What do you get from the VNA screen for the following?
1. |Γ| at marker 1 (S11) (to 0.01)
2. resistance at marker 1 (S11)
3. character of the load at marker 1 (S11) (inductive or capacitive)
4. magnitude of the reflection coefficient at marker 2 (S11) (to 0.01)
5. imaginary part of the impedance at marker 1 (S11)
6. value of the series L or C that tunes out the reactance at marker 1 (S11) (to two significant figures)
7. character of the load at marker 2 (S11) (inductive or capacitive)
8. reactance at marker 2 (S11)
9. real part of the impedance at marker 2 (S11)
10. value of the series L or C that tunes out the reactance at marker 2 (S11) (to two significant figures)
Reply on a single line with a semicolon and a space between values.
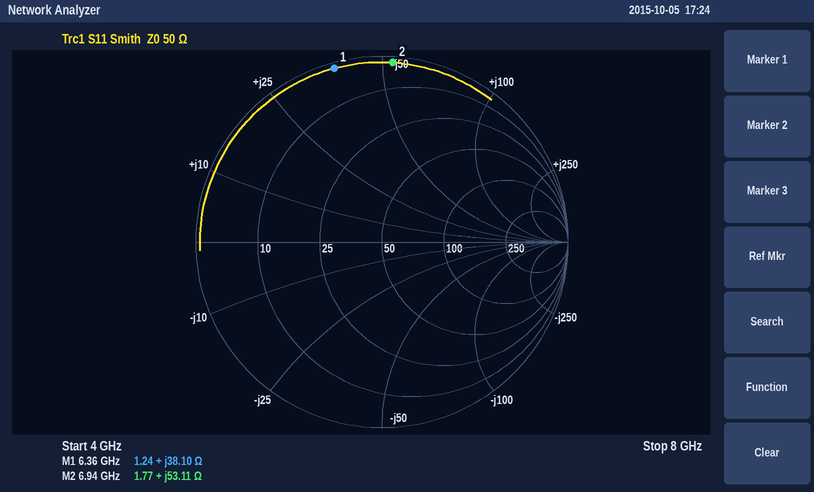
0.97; 1.24 Ω; inductive; 0.97; +38.10 Ω; 660 fF; inductive; +53.11 Ω; 1.77 Ω; 430 fF
